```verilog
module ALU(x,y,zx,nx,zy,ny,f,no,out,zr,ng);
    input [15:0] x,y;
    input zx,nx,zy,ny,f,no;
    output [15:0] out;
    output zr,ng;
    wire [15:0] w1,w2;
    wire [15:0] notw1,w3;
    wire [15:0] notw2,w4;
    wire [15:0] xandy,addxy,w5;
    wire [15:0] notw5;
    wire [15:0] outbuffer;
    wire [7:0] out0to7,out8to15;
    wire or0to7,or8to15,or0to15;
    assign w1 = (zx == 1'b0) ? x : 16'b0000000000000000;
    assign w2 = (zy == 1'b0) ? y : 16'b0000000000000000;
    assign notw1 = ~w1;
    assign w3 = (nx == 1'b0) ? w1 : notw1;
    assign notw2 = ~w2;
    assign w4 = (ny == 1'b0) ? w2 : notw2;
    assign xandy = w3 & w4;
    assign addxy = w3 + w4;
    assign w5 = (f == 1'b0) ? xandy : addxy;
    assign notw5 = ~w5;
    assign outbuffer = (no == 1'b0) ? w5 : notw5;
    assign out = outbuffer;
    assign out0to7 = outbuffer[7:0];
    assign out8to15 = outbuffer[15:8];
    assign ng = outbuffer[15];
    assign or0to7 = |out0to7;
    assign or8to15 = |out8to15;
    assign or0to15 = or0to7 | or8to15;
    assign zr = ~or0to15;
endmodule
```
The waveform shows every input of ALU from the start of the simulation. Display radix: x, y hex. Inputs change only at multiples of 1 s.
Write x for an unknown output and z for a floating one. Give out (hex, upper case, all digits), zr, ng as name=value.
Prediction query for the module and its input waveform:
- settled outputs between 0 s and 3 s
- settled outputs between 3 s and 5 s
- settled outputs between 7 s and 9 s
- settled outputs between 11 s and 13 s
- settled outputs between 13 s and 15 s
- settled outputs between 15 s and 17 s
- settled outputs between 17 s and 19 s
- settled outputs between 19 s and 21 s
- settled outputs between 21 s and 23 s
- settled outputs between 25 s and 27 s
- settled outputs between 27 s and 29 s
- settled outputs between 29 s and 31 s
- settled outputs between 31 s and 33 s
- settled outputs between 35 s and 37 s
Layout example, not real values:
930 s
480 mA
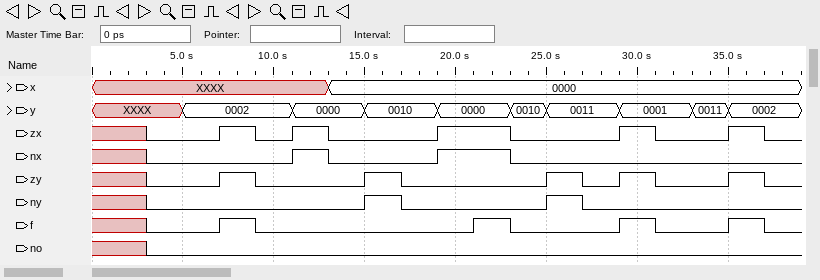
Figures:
out=x, zr=x, ng=x
out=x, zr=x, ng=x
out=0000, zr=1, ng=0
out=0000, zr=1, ng=0
out=0000, zr=1, ng=0
out=0000, zr=1, ng=0
out=0000, zr=1, ng=0
out=0000, zr=1, ng=0
out=FFFF, zr=0, ng=1
out=0000, zr=1, ng=0
out=0000, zr=1, ng=0
out=0000, zr=1, ng=0
out=0000, zr=1, ng=0
out=0000, zr=1, ng=0
